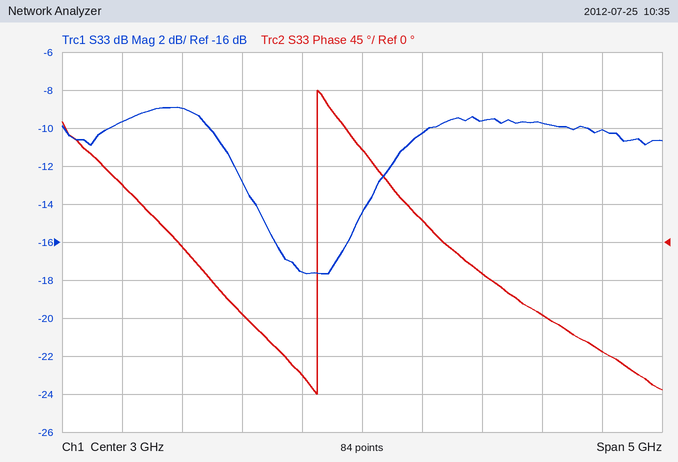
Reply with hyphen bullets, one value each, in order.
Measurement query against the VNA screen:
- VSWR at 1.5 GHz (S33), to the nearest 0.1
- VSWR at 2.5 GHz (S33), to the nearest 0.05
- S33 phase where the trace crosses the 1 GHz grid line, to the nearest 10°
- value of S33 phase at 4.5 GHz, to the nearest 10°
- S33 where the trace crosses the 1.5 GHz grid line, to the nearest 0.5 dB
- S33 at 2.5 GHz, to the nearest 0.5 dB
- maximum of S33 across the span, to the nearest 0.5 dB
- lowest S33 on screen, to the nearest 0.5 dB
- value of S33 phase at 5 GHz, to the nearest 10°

- 2.1
- 1.30
- 70°
- -90°
- -9.0 dB
- -17.5 dB
- -9.0 dB
- -17.5 dB
- -130°
